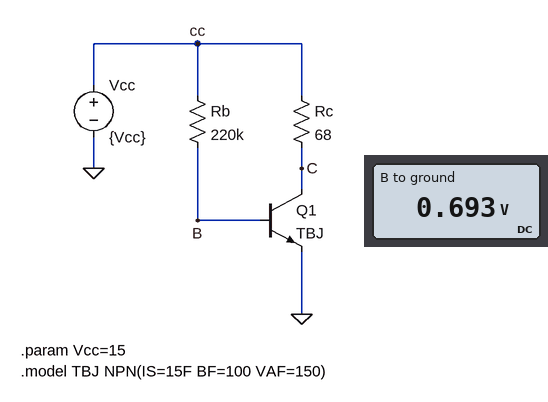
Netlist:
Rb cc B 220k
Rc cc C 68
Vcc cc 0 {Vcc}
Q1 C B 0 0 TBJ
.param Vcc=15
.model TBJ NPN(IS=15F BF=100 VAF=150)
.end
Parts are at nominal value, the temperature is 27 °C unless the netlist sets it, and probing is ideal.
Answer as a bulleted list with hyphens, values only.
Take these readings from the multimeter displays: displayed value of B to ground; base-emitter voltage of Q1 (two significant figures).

- 0.693 V
- 690 mV
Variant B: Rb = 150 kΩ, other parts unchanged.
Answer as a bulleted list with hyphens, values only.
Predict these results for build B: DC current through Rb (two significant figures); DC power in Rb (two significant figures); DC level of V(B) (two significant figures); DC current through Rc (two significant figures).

- 95 µA
- 1.4 mW
- 700 mV
- 10 mA
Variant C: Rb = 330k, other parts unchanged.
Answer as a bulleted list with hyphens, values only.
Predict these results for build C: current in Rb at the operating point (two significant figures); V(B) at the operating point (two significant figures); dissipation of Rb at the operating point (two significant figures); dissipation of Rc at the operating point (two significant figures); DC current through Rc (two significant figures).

- 43 µA
- 680 mV
- 620 µW
- 1.5 mW
- 4.7 mA
